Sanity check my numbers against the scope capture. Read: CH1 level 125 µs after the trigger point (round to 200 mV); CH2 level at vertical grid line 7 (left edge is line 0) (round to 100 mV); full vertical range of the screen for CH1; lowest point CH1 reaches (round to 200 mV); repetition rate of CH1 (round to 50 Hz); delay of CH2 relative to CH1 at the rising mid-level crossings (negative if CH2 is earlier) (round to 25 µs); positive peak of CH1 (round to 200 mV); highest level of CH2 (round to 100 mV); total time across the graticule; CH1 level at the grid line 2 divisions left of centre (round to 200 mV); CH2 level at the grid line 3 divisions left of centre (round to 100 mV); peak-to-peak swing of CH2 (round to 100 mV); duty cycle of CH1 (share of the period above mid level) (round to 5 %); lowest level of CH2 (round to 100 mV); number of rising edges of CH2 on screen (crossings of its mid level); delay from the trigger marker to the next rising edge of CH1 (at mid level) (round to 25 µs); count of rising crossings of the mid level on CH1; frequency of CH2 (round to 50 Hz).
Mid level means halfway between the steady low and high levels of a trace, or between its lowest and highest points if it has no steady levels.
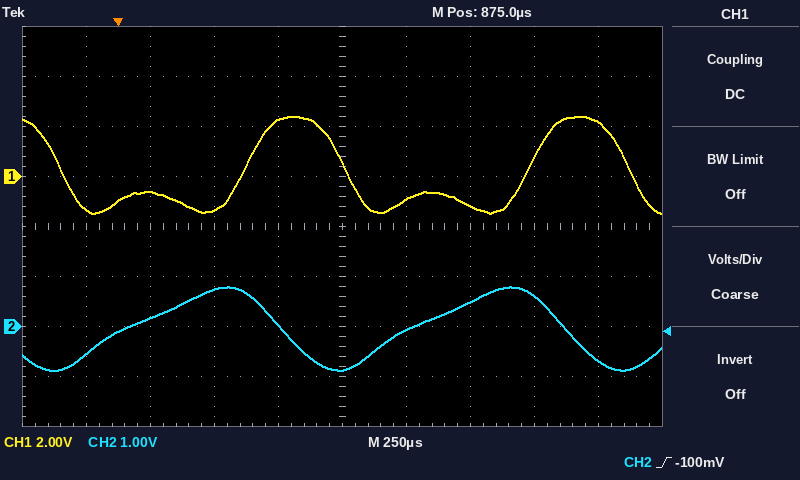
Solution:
-600 mV
500 mV
16 V
-1.4 V
900 Hz
-475 µs
2.4 V
800 mV
2.5 ms
-1.4 V
200 mV
1.7 V
35 %
-900 mV
2
500 µs
2
900 Hz
